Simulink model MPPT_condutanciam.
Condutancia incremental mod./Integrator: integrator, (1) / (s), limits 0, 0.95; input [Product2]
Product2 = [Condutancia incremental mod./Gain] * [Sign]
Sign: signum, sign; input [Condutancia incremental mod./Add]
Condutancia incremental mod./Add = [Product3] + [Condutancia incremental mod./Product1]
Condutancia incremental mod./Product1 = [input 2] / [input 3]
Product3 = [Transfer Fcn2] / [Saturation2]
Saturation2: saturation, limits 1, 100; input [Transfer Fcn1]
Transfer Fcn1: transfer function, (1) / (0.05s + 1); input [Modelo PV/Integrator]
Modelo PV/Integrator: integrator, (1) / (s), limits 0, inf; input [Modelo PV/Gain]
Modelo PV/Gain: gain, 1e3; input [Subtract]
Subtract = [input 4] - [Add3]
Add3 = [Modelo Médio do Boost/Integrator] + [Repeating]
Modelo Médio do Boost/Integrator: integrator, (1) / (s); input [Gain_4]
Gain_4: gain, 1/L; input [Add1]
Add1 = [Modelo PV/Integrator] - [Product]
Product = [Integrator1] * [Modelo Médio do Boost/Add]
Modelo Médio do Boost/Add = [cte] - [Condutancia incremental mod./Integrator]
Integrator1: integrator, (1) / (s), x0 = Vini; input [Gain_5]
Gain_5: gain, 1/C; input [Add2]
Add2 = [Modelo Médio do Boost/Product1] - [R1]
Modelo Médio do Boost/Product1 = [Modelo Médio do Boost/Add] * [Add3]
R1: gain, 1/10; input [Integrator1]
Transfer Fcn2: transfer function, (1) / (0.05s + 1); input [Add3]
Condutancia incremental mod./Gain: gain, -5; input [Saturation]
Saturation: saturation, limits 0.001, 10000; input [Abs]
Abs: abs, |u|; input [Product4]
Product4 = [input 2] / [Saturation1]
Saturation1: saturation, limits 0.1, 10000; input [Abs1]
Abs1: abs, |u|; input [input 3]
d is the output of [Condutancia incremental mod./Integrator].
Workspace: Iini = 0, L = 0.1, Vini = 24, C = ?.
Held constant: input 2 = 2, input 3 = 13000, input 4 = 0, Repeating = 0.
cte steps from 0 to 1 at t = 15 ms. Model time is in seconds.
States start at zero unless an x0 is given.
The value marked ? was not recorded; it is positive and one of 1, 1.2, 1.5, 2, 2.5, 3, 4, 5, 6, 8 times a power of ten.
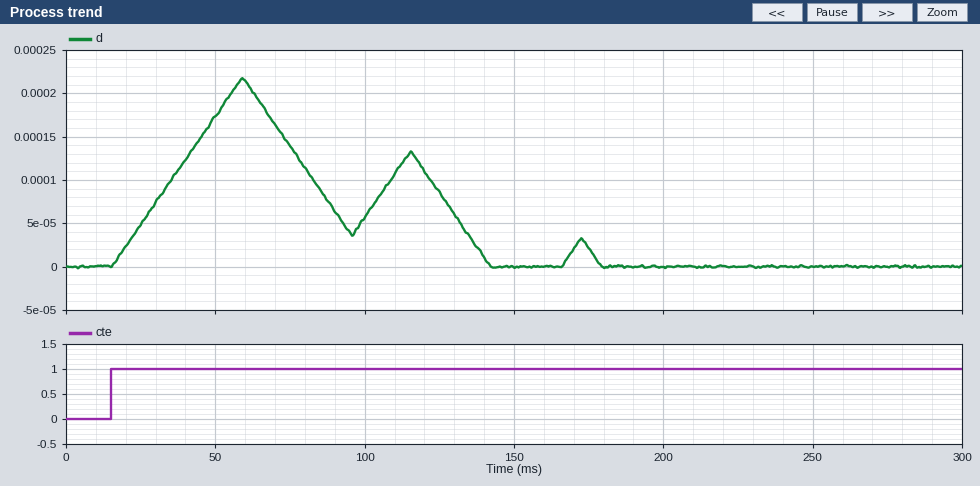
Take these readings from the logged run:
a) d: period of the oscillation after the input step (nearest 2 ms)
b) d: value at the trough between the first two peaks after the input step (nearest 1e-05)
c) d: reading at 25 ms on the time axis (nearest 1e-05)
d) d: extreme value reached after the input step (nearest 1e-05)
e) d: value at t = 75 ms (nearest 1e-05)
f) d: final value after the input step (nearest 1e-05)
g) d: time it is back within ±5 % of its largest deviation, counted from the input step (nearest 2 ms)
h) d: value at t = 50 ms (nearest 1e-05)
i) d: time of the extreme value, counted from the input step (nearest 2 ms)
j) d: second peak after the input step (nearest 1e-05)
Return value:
56 ms
0.00004
0.00005
0.00022
0.00014
0.00000
162 ms
0.00017
44 ms
0.00013
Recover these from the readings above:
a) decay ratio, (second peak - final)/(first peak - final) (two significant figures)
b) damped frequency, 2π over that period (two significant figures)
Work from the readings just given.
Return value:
0.59
0.11 rad/ms
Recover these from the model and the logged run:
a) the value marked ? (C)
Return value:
0.01
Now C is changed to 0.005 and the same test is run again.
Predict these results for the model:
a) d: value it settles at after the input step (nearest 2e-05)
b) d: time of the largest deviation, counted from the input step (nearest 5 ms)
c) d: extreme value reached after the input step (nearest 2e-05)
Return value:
0.00000
40 ms
0.00020
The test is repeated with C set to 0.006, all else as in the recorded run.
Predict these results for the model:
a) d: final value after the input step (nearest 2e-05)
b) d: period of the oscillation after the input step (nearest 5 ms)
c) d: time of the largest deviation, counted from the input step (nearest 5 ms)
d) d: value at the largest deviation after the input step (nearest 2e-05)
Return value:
0.00000
50 ms
40 ms
0.00020
